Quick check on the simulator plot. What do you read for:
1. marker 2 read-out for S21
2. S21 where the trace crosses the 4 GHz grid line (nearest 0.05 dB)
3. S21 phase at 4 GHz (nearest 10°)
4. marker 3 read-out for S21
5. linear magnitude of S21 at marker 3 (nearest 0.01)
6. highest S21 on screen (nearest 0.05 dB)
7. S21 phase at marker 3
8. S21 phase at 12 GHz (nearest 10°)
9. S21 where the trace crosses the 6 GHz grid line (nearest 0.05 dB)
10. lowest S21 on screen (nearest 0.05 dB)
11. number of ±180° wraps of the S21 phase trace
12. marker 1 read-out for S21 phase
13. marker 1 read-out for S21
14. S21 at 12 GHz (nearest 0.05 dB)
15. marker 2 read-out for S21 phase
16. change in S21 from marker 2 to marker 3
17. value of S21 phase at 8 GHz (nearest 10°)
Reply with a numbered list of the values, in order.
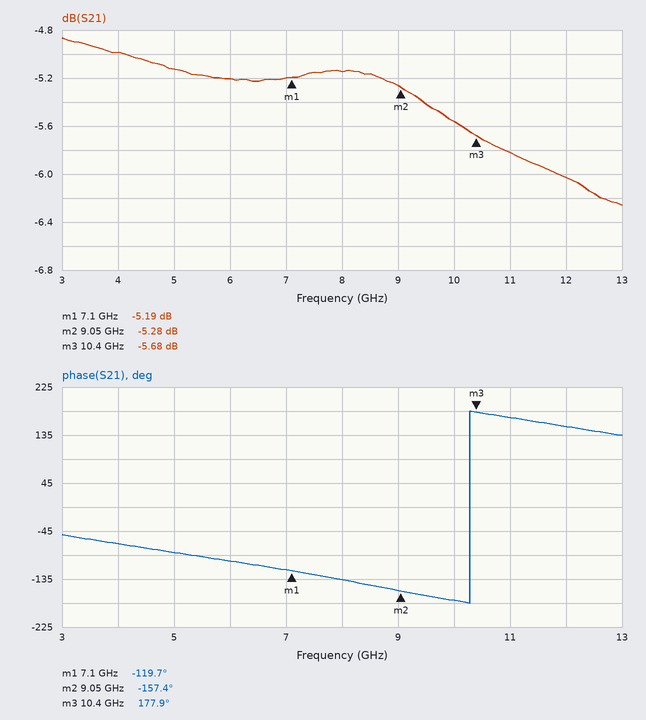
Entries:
1. -5.28 dB
2. -5.00 dB
3. -70°
4. -5.68 dB
5. 0.52
6. -4.85 dB
7. 177.9°
8. 150°
9. -5.20 dB
10. -6.25 dB
11. 1
12. -119.7°
13. -5.19 dB
14. -6.05 dB
15. -157.4°
16. -0.40 dB
17. -140°
